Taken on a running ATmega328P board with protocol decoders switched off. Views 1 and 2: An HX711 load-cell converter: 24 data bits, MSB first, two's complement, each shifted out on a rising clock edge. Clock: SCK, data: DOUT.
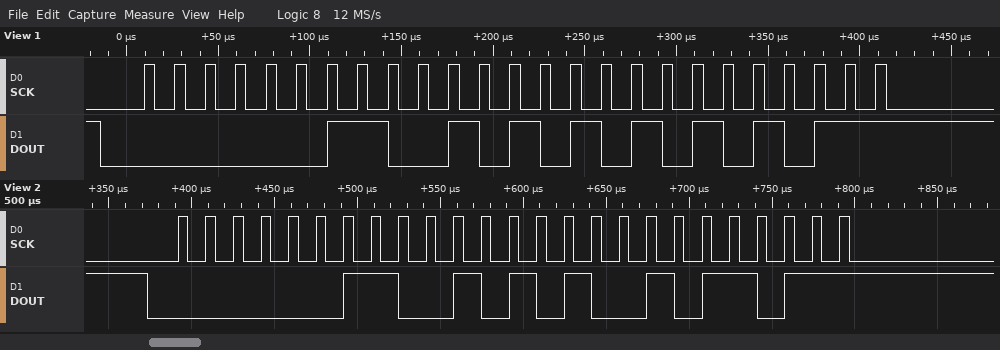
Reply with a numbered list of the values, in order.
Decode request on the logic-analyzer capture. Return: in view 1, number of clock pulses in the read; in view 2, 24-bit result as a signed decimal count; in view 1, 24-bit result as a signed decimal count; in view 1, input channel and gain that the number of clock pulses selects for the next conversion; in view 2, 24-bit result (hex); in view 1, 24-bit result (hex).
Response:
1. 25
2. 207451
3. 207531
4. channel A, gain 128
5. 0x032A5B
6. 0x032AAB
